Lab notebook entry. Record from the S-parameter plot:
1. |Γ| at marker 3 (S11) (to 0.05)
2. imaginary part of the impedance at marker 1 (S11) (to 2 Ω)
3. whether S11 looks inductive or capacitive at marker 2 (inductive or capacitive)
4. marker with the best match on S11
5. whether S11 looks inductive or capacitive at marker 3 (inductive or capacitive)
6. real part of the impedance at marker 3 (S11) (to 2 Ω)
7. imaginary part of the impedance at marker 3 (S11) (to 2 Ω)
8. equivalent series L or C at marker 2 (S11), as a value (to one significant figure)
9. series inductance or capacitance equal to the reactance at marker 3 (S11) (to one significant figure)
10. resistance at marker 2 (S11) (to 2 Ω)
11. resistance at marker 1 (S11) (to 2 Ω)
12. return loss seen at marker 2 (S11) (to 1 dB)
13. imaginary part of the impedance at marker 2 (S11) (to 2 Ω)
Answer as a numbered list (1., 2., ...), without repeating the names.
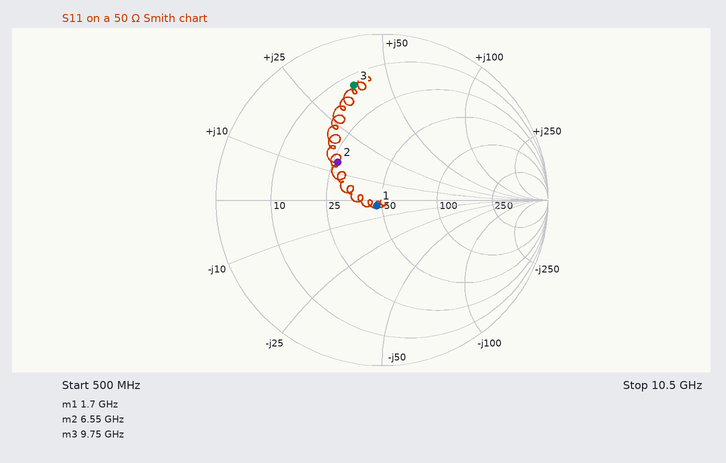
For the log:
1. 0.70
2. -4 Ω
3. inductive
4. marker 1
5. inductive
6. 14 Ω
7. +38 Ω
8. 300 pH
9. 600 pH
10. 26 Ω
11. 46 Ω
12. 9 dB
13. +14 Ω
